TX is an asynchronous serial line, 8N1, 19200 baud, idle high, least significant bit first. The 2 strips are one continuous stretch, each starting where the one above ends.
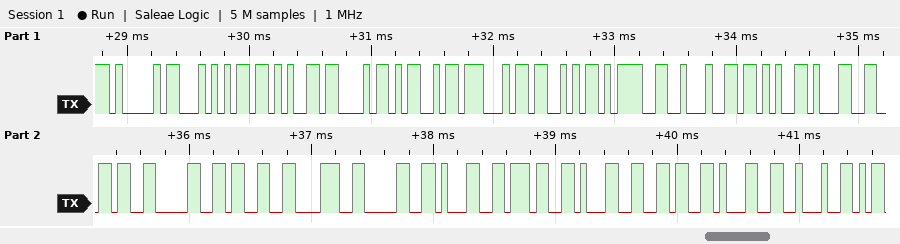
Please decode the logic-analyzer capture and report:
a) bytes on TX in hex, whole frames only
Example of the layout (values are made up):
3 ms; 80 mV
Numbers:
41 54 2B 43 4D 47 53 3D 22 2B 31 36 30 33 38 30 31 37 31 36 31 22
